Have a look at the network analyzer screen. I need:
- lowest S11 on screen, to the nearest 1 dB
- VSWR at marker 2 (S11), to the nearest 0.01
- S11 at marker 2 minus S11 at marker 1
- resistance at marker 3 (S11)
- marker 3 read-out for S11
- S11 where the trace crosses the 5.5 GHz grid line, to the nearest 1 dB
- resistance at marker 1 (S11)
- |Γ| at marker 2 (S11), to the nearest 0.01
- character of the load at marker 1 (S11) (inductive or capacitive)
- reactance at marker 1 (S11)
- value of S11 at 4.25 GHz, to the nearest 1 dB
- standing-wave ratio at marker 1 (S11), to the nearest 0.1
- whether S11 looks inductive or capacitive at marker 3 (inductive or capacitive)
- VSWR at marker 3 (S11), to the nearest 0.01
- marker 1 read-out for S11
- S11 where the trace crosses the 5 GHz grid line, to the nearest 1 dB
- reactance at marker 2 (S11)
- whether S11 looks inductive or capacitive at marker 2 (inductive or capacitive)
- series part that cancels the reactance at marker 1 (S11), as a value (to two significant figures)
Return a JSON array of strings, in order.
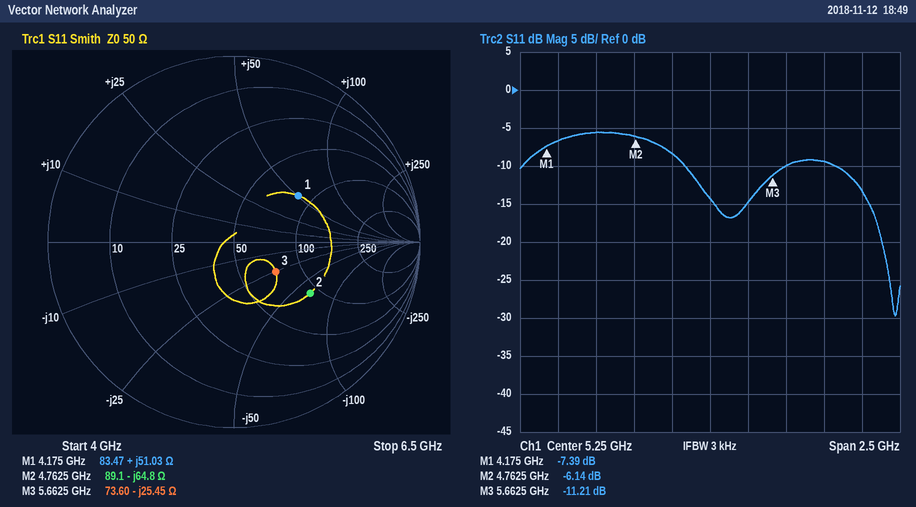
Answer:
["-30 dB", "2.95", "1.25 dB", "73.60 Ω", "-11.21 dB", "-15 dB", "83.47 Ω", "0.49", "inductive", "+51.03 Ω", "-7 dB", "2.5", "capacitive", "1.76", "-7.39 dB", "-8 dB", "-64.8 Ω", "capacitive", "750 fF"]
